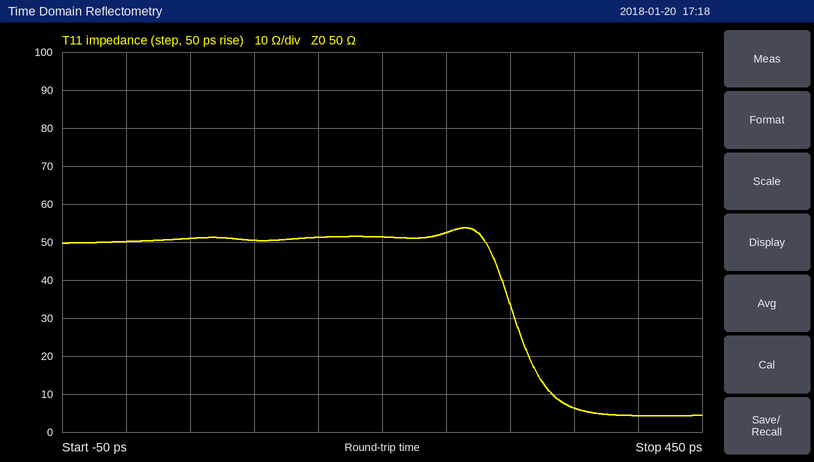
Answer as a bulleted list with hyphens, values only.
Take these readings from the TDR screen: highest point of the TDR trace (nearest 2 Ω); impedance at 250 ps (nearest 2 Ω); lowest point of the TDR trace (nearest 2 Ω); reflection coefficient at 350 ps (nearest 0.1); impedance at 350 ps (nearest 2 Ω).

- 54 Ω
- 52 Ω
- 4 Ω
- -0.8
- 6 Ω
